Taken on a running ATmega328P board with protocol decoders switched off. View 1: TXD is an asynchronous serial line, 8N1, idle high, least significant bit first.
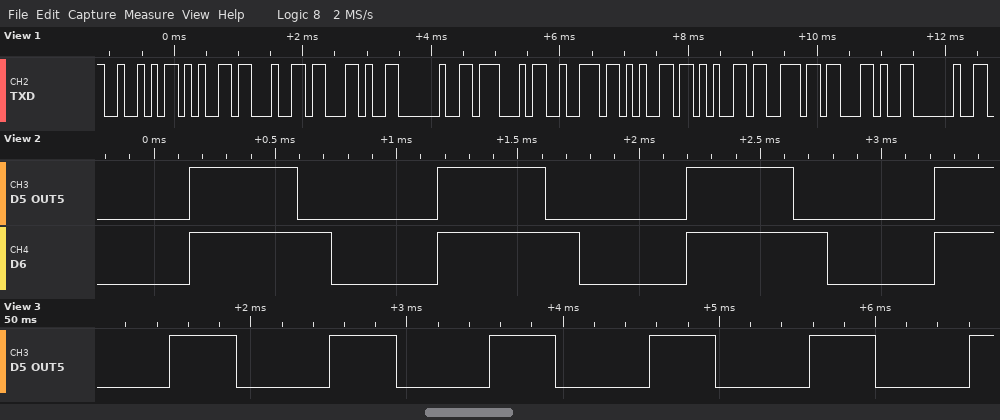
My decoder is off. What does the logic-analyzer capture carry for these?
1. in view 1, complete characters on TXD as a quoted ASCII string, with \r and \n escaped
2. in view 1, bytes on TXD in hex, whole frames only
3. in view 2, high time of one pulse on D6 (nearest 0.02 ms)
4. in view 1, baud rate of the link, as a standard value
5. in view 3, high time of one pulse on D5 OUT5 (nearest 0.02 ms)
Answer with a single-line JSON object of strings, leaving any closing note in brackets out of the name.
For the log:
{"in view 1, complete characters on TXD as a quoted ASCII string, with \\r and \\n escaped": "\"Red, Green, \"", "in view 1, bytes on TXD in hex, whole frames only": "52 65 64 2C 20 47 72 65 65 6E 2C 20", "in view 2, high time of one pulse on D6": "0.58 ms", "in view 1, baud rate of the link, as a standard value": "9600 baud", "in view 3, high time of one pulse on D5 OUT5": "0.42 ms"}
